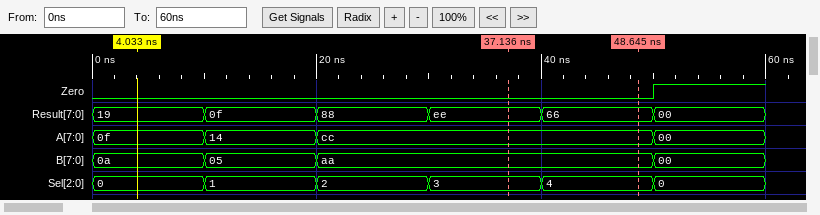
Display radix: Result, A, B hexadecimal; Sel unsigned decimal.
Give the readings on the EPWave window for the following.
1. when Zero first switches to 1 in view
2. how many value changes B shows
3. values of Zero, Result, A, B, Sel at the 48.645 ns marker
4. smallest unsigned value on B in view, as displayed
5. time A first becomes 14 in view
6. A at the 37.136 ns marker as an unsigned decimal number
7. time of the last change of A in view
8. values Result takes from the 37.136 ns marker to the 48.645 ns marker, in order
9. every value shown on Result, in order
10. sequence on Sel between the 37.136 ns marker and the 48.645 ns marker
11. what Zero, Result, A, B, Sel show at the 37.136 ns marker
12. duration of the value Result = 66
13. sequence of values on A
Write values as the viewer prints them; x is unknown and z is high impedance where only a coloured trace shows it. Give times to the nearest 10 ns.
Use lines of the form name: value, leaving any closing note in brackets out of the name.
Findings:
when Zero first switches to 1 in view: 50 ns
how many value changes B shows: 3
values of Zero, Result, A, B, Sel at the 48.645 ns marker: Zero=0, Result=66, A=cc, B=aa, Sel=4
smallest unsigned value on B in view, as displayed: 00
time A first becomes 14 in view: 10 ns
A at the 37.136 ns marker as an unsigned decimal number: 204
time of the last change of A in view: 50 ns
values Result takes from the 37.136 ns marker to the 48.645 ns marker, in order: ee, 66
every value shown on Result, in order: 19, 0f, 88, ee, 66, 00
sequence on Sel between the 37.136 ns marker and the 48.645 ns marker: 3, 4
what Zero, Result, A, B, Sel show at the 37.136 ns marker: Zero=0, Result=ee, A=cc, B=aa, Sel=3
duration of the value Result = 66: 10 ns
sequence of values on A: 0f, 14, cc, 00
